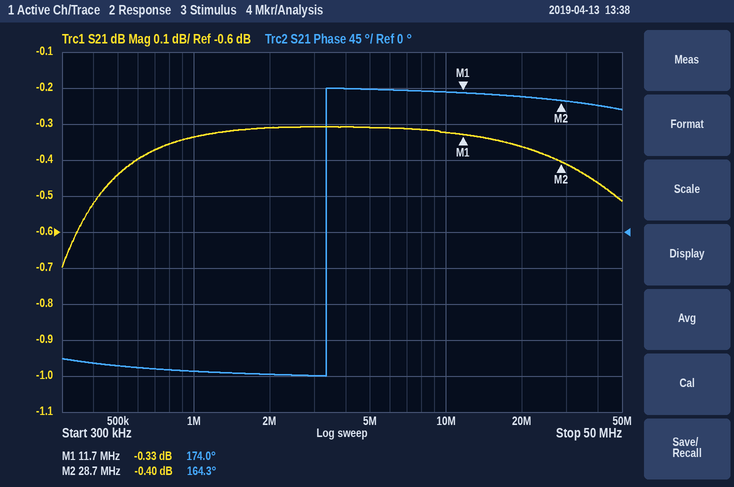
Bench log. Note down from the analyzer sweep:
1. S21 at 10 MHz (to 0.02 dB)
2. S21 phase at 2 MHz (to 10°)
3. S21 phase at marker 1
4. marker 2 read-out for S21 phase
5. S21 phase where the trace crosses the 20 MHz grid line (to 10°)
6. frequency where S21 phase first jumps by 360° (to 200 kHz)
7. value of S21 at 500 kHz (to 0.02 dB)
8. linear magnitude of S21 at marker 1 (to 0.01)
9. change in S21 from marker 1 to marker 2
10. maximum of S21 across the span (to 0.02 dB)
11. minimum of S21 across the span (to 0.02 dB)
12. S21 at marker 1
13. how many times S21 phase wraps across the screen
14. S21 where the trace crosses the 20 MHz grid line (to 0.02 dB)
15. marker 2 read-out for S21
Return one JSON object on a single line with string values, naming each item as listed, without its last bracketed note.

{"S21 at 10 MHz": "-0.32 dB", "S21 phase at 2 MHz": "-180°", "S21 phase at marker 1": "174.0°", "marker 2 read-out for S21 phase": "164.3°", "S21 phase where the trace crosses the 20 MHz grid line": "170°", "frequency where S21 phase first jumps by 360°": "3.4 MHz", "value of S21 at 500 kHz": "-0.44 dB", "linear magnitude of S21 at marker 1": "0.96", "change in S21 from marker 1 to marker 2": "-0.07 dB", "maximum of S21 across the span": "-0.30 dB", "minimum of S21 across the span": "-0.70 dB", "S21 at marker 1": "-0.33 dB", "how many times S21 phase wraps across the screen": "1", "S21 where the trace crosses the 20 MHz grid line": "-0.36 dB", "marker 2 read-out for S21": "-0.40 dB"}
